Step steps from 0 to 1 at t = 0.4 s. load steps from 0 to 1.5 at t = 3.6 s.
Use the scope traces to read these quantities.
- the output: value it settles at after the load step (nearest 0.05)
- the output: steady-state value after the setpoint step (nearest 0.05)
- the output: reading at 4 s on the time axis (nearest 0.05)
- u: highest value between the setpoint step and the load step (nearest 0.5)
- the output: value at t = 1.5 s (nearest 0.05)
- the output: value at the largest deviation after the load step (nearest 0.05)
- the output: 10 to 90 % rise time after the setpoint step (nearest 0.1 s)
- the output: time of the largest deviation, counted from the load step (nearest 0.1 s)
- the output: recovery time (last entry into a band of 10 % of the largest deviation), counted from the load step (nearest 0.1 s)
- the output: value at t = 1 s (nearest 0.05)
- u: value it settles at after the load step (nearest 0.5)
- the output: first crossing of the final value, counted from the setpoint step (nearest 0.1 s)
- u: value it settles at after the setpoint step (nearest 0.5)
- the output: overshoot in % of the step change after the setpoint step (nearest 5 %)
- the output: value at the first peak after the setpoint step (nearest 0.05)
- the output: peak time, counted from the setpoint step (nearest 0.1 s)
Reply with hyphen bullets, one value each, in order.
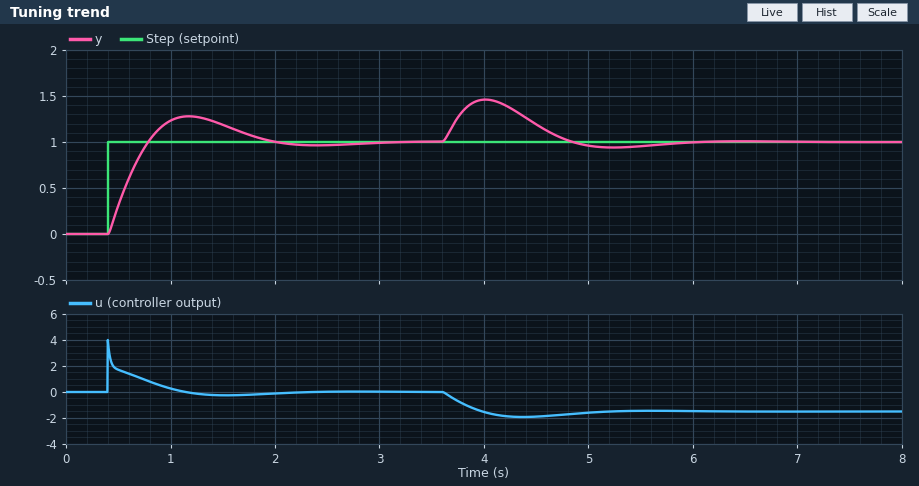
- 1.00
- 1.00
- 1.45
- 4.0
- 1.20
- 1.45
- 0.3 s
- 0.4 s
- 1.9 s
- 1.25
- -1.5
- 0.4 s
- 0.0
- 30 %
- 1.30
- 0.8 s
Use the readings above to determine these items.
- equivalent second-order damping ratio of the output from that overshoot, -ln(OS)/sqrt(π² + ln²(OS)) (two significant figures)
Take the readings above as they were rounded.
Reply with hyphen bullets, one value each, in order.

- 0.36
